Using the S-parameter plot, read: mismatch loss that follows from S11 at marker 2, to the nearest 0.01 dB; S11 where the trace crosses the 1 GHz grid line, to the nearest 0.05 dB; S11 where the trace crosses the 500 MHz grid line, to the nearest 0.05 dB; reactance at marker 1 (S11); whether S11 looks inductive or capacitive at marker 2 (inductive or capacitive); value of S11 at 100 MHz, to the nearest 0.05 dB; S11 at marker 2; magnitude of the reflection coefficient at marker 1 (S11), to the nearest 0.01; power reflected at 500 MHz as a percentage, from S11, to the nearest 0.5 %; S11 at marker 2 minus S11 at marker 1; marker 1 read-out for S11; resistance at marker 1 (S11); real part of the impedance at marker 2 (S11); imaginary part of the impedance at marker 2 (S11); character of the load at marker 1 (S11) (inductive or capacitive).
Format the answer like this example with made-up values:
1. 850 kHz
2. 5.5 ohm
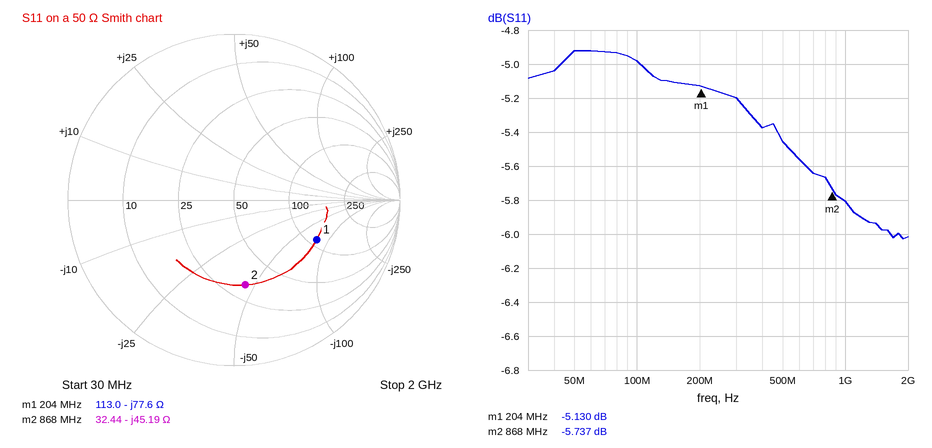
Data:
1. 1.35 dB
2. -5.80 dB
3. -5.45 dB
4. -77.6 Ω
5. capacitive
6. -5.00 dB
7. -5.737 dB
8. 0.55
9. 28.5 %
10. -0.607 dB
11. -5.130 dB
12. 113.0 Ω
13. 32.44 Ω
14. -45.19 Ω
15. capacitive
